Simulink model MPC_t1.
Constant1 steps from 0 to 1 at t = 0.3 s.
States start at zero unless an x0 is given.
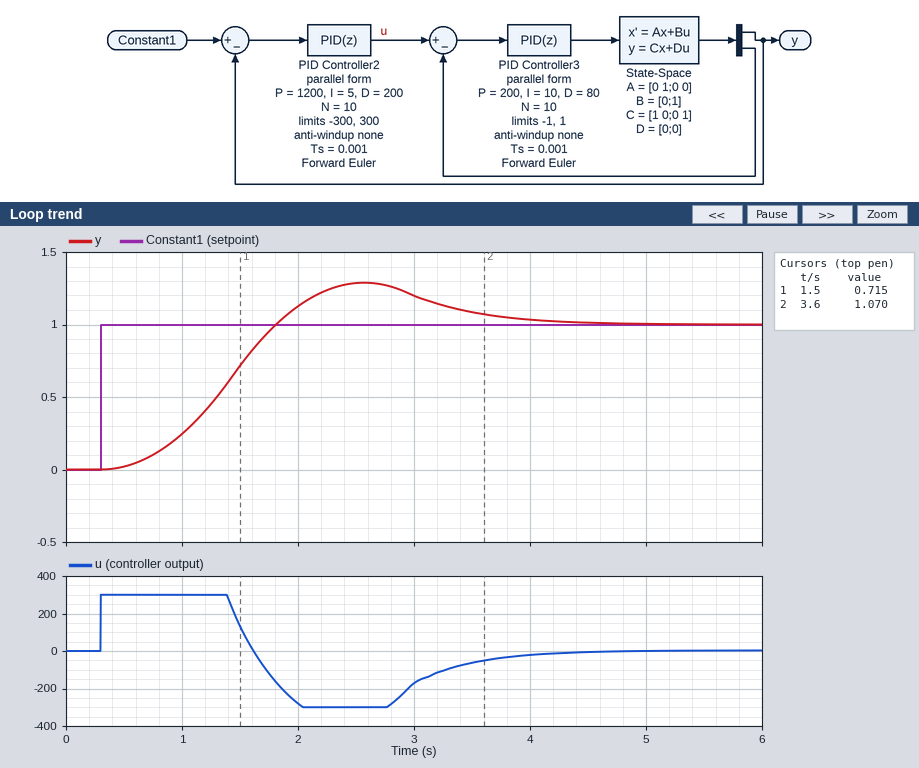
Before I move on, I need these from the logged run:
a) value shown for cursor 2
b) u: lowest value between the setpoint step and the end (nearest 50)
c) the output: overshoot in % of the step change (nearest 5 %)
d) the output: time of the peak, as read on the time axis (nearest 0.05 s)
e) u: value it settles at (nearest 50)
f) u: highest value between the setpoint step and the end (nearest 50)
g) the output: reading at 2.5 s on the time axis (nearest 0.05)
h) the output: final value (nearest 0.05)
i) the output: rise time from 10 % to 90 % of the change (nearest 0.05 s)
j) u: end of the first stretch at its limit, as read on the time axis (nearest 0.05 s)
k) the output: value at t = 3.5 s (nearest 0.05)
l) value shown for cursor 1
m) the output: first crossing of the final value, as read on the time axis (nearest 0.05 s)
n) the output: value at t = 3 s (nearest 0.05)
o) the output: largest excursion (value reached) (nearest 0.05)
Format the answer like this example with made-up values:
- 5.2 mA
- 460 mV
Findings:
- 1.070
- -300
- 30 %
- 2.55 s
- 0
- 300
- 1.30
- 1.00
- 0.95 s
- 1.40 s
- 1.10
- 0.715
- 1.80 s
- 1.20
- 1.30
